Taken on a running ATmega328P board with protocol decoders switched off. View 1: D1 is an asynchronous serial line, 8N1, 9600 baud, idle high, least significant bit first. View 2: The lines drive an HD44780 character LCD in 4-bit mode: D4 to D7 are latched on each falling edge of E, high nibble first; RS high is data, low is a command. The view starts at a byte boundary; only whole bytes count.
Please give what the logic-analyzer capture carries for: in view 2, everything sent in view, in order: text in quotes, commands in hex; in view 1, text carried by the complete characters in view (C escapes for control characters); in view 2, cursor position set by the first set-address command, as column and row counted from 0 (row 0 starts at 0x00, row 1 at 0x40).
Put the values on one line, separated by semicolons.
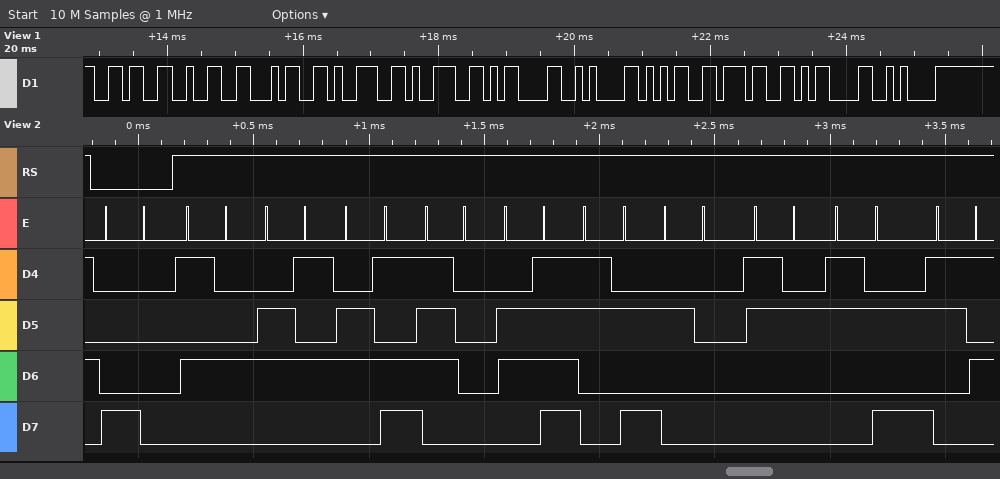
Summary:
0x80 "Tempo: 2:5"; "62499\r\n57\r\n"; column 0, row 0
